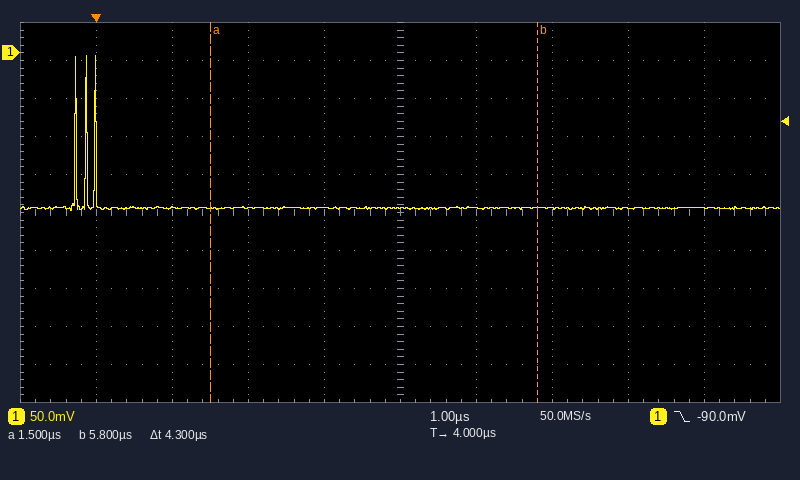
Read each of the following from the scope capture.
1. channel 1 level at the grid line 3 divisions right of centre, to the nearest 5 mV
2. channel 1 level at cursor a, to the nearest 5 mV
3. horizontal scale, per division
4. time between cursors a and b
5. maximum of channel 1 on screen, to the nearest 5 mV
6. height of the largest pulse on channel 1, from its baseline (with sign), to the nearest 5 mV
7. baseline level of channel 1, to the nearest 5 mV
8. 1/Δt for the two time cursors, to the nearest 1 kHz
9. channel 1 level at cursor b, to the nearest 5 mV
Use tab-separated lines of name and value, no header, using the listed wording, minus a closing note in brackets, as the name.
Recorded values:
channel 1 level at the grid line 3 divisions right of centre, to the nearest 5 mV	-205 mV
channel 1 level at cursor a, to the nearest 5 mV	-205 mV
horizontal scale, per division	1 µs
time between cursors a and b	4.3 µs
maximum of channel 1 on screen, to the nearest 5 mV	-5 mV
height of the largest pulse on channel 1, from its baseline (with sign), to the nearest 5 mV	+200 mV
baseline level of channel 1, to the nearest 5 mV	-205 mV
1/Δt for the two time cursors, to the nearest 1 kHz	233 kHz
channel 1 level at cursor b, to the nearest 5 mV	-205 mV
